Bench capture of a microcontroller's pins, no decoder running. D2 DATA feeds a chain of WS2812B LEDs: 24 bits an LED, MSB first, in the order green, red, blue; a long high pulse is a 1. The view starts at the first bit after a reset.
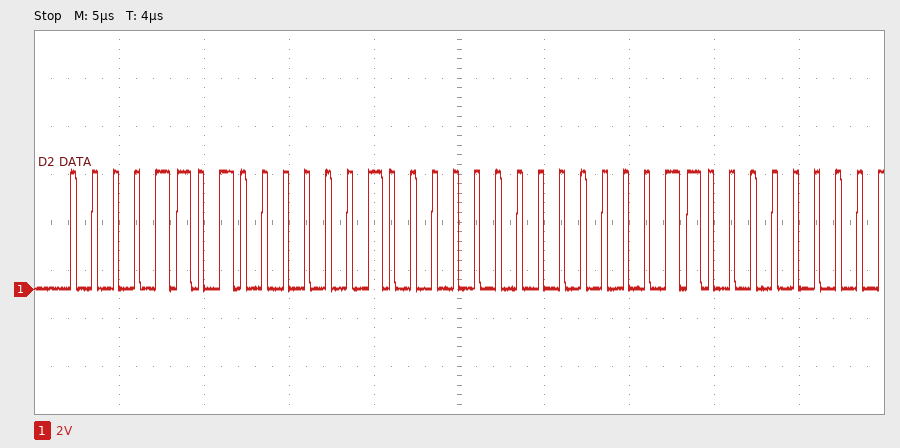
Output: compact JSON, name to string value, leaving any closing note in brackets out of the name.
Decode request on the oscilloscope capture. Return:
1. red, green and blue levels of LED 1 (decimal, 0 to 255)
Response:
{"red, green and blue levels of LED 1": "2, 13, 0"}
